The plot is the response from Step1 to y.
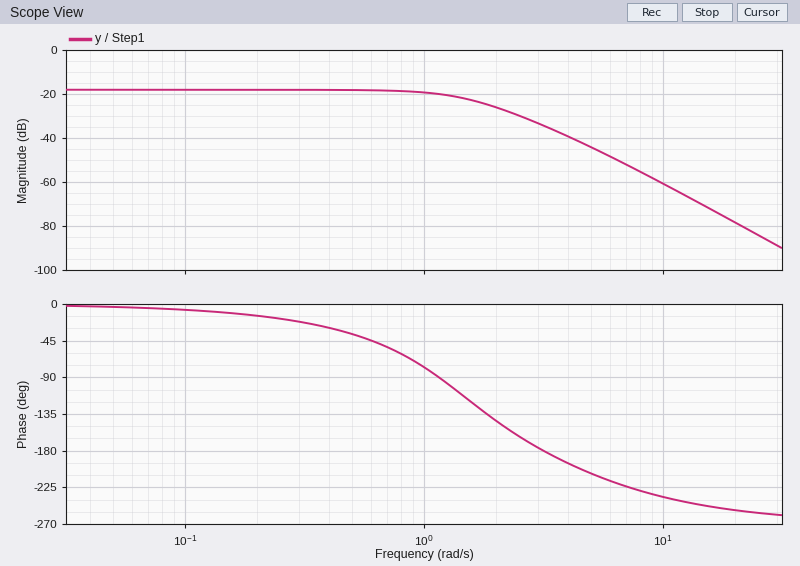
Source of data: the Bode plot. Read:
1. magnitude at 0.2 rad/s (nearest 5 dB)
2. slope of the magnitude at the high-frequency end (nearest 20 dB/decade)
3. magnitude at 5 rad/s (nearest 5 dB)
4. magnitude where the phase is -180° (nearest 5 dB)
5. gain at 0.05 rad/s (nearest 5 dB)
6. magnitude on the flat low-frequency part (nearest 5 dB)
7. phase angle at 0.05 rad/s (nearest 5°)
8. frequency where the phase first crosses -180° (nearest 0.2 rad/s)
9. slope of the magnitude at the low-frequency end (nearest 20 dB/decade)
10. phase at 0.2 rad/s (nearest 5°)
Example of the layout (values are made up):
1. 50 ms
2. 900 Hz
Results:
1. -20 dB
2. -60 dB/decade
3. -45 dB
4. -35 dB
5. -20 dB
6. -20 dB
7. -5°
8. 3.2 rad/s
9. 0 dB/decade
10. -15°
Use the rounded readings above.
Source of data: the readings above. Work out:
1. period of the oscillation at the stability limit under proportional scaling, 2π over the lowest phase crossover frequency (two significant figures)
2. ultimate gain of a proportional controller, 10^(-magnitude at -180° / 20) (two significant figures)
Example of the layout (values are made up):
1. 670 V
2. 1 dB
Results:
1. 2.0 s
2. 56
